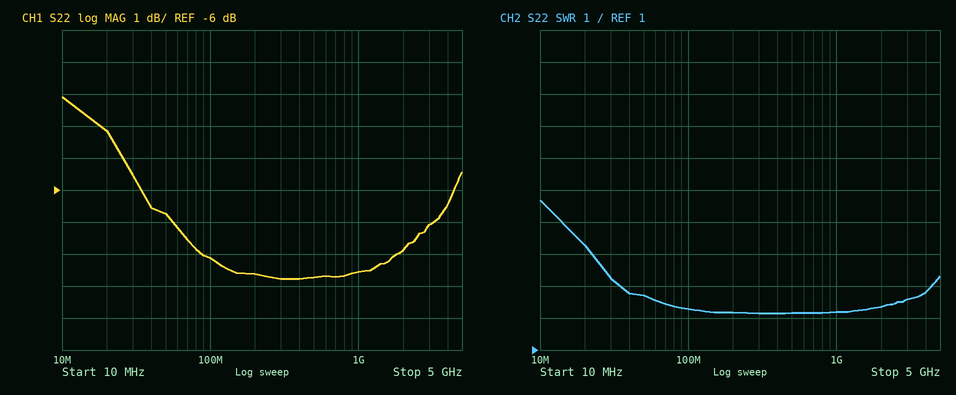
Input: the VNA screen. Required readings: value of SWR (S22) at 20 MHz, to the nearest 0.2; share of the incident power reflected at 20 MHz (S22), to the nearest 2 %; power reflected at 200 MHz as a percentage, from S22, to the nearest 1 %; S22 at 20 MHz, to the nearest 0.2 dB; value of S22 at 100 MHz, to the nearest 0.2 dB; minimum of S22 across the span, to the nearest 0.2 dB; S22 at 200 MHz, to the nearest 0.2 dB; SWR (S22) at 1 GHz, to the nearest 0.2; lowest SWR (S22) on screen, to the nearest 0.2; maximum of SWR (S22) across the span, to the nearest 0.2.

4.2
38 %
14 %
-4.2 dB
-8.2 dB
-8.8 dB
-8.6 dB
2.2
2.2
5.6
